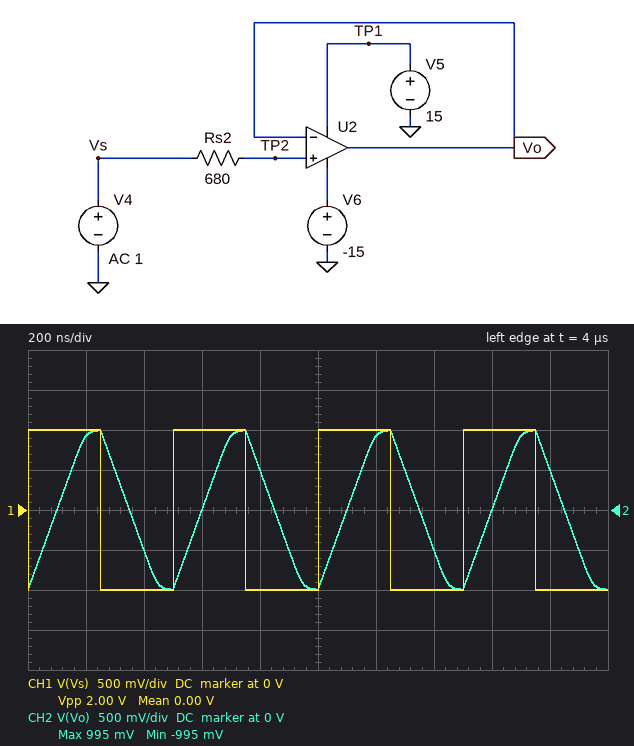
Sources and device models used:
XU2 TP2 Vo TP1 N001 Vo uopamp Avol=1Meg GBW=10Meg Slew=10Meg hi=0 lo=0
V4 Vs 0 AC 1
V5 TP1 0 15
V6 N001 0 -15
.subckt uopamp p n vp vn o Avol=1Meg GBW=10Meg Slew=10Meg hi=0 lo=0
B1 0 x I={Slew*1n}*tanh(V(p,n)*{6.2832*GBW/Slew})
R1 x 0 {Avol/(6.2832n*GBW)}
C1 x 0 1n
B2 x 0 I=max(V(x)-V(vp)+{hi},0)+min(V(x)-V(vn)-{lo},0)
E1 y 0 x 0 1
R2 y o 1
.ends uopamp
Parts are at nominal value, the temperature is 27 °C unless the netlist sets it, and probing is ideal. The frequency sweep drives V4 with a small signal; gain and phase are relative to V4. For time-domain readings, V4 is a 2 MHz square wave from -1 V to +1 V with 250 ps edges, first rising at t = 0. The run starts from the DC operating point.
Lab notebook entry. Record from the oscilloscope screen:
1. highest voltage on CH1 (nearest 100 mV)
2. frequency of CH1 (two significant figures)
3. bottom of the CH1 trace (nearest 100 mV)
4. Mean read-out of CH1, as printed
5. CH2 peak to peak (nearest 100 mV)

1.0 V
2.0 MHz
-1.0 V
0.00 V
2.0 V
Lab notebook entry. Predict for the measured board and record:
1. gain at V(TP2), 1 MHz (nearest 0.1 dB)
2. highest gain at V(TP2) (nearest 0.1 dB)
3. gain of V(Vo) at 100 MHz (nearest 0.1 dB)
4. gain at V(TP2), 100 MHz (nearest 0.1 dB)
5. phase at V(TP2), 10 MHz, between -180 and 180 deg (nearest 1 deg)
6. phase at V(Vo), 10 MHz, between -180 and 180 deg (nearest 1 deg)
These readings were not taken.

0 dB
0 dB
-20.0 dB
0 dB
0 deg
-45 deg
